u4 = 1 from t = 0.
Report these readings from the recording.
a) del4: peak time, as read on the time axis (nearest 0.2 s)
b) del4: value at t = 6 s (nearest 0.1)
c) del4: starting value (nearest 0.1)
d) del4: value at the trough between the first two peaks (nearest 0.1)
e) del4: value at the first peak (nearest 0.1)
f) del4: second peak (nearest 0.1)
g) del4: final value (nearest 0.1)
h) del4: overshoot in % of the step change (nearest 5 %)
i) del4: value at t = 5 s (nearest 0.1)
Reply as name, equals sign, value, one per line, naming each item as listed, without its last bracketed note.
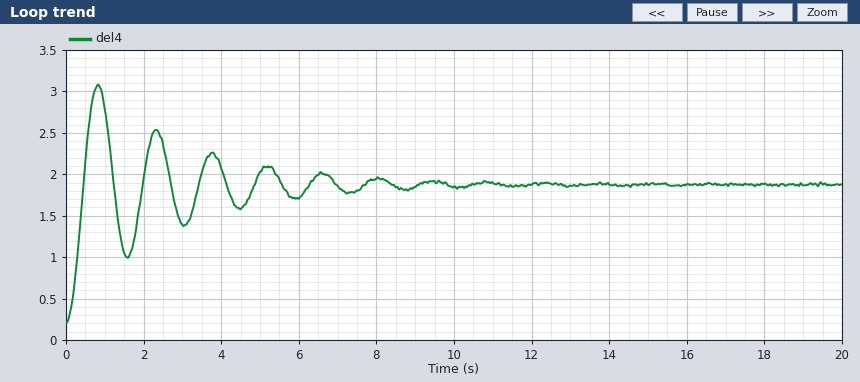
del4: peak time, as read on the time axis = 0.8 s
del4: value at t = 6 s = 1.7
del4: starting value = 0.2
del4: value at the trough between the first two peaks = 1.0
del4: value at the first peak = 3.1
del4: second peak = 2.5
del4: final value = 1.9
del4: overshoot in % of the step change = 70 %
del4: value at t = 5 s = 2.0
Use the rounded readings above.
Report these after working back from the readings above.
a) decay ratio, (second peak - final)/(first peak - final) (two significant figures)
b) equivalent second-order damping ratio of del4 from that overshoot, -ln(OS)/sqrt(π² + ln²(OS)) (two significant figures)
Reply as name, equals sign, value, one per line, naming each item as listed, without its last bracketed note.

decay ratio, (second peak - final)/(first peak - final) = 0.50
equivalent second-order damping ratio of del4 from that overshoot, -ln(OS)/sqrt(π² + ln²(OS)) = 0.11
